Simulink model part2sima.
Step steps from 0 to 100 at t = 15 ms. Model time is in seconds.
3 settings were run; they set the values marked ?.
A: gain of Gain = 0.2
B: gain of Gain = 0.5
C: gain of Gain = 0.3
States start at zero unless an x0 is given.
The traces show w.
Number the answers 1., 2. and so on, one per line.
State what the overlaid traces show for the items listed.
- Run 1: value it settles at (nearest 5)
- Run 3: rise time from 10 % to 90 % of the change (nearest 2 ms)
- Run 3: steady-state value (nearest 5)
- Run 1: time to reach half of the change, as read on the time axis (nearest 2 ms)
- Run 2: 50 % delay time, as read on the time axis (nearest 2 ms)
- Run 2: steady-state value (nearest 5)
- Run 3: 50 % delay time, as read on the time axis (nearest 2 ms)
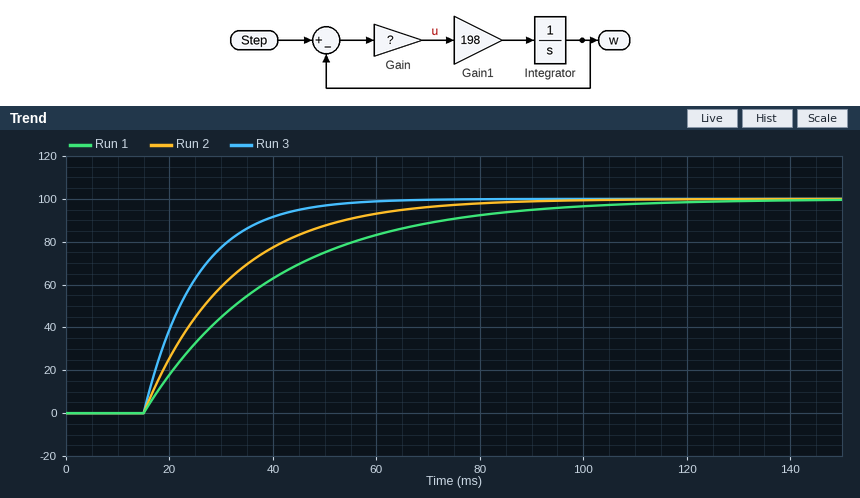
1. 100
2. 22 ms
3. 100
4. 32 ms
5. 26 ms
6. 100
7. 22 ms
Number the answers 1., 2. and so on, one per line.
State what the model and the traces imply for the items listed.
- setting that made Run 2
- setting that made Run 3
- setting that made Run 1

1. C
2. B
3. A
